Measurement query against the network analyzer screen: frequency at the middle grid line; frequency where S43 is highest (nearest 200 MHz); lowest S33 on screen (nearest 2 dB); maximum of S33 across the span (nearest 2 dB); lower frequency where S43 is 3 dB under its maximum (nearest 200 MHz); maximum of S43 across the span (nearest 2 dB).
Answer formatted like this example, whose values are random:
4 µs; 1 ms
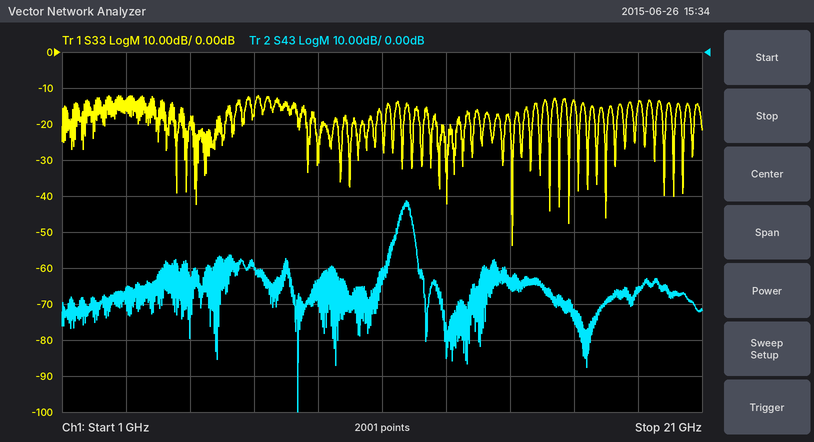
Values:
11 GHz; 11.8 GHz; -54 dB; -12 dB; 11.6 GHz; -42 dB
